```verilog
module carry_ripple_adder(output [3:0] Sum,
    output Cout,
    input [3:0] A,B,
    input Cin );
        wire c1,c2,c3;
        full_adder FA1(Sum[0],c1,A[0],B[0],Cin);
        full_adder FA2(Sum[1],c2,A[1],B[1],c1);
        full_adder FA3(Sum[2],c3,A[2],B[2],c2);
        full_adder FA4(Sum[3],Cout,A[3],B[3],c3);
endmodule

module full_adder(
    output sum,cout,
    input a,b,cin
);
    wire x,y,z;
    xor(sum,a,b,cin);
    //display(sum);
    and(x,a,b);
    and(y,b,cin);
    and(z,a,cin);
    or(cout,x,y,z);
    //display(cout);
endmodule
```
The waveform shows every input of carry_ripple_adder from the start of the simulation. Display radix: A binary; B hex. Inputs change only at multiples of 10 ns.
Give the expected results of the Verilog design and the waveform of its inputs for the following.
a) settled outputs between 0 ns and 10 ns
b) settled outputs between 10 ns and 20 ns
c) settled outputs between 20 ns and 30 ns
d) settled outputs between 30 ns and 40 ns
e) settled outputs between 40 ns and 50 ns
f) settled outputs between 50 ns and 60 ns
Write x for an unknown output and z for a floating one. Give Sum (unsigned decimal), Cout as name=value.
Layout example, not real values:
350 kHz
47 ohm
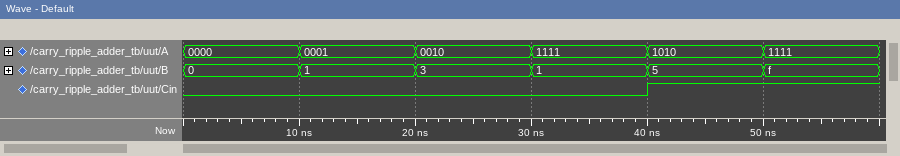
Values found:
Sum=0, Cout=0
Sum=2, Cout=0
Sum=5, Cout=0
Sum=0, Cout=1
Sum=0, Cout=1
Sum=15, Cout=1
